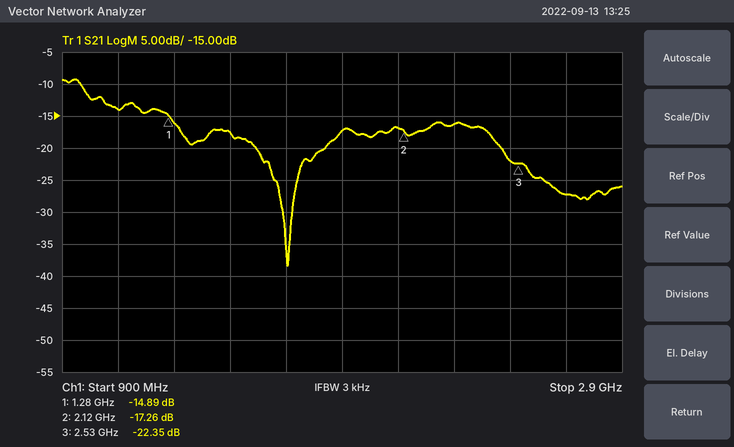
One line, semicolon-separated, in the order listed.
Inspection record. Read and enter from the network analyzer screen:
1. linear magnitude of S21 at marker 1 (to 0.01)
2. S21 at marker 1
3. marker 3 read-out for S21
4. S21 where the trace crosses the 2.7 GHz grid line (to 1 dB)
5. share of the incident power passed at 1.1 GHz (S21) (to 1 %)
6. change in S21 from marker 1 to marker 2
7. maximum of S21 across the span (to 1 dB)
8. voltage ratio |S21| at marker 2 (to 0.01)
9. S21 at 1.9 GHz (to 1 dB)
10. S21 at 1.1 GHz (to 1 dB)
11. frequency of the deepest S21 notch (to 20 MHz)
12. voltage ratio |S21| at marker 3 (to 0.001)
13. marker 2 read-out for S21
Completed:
0.18; -14.89 dB; -22.35 dB; -27 dB; 4 %; -2.37 dB; -9 dB; 0.14; -17 dB; -14 dB; 1.70 GHz; 0.076; -17.26 dB
